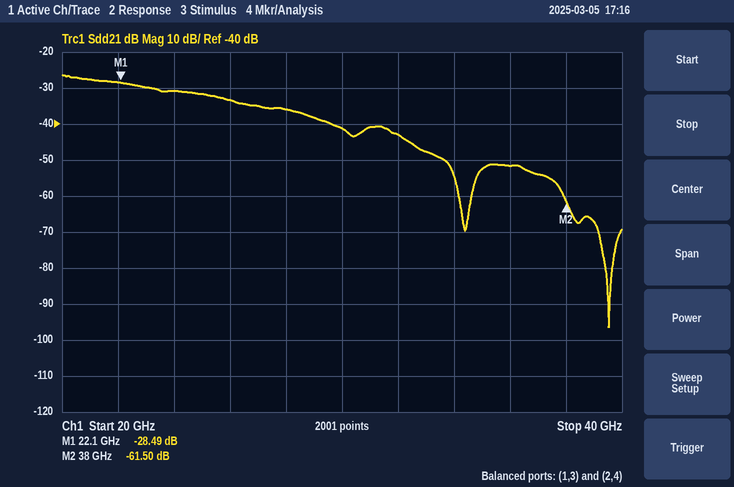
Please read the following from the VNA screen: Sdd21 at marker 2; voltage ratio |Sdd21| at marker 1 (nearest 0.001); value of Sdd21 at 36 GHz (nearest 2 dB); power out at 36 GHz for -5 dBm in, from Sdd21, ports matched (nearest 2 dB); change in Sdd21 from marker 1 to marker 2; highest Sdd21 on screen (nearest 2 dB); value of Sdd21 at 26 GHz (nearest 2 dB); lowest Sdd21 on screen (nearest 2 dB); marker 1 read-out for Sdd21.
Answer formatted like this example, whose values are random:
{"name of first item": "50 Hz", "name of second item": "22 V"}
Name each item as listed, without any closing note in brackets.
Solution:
{"Sdd21 at marker 2": "-61.50 dB", "voltage ratio |Sdd21| at marker 1": "0.038", "value of Sdd21 at 36 GHz": "-52 dB", "power out at 36 GHz for -5 dBm in, from Sdd21, ports matched": "-56 dBm", "change in Sdd21 from marker 1 to marker 2": "-33.01 dB", "highest Sdd21 on screen": "-26 dB", "value of Sdd21 at 26 GHz": "-34 dB", "lowest Sdd21 on screen": "-96 dB", "marker 1 read-out for Sdd21": "-28.49 dB"}
